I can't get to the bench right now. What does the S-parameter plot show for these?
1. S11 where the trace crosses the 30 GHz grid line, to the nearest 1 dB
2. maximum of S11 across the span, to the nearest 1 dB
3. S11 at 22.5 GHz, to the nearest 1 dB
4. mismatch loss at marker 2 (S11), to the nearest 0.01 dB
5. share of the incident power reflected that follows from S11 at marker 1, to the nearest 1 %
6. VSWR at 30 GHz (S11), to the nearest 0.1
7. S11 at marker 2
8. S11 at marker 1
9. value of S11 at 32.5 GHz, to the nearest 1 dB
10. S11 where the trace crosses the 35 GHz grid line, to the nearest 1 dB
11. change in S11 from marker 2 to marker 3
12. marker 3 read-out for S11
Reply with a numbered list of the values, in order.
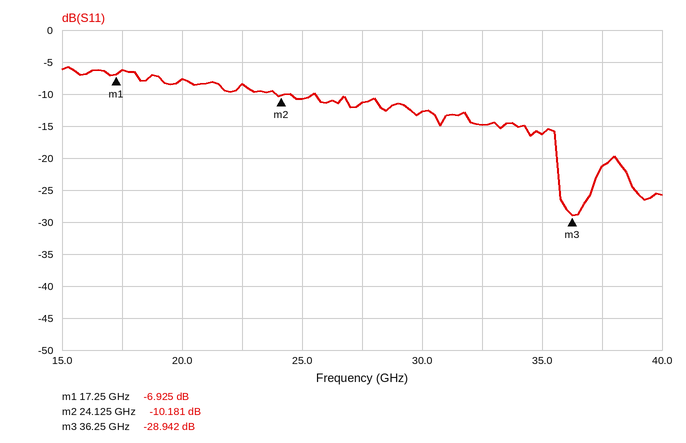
1. -13 dB
2. -6 dB
3. -8 dB
4. 0.44 dB
5. 20 %
6. 1.6
7. -10.181 dB
8. -6.925 dB
9. -15 dB
10. -16 dB
11. -18.761 dB
12. -28.942 dB
